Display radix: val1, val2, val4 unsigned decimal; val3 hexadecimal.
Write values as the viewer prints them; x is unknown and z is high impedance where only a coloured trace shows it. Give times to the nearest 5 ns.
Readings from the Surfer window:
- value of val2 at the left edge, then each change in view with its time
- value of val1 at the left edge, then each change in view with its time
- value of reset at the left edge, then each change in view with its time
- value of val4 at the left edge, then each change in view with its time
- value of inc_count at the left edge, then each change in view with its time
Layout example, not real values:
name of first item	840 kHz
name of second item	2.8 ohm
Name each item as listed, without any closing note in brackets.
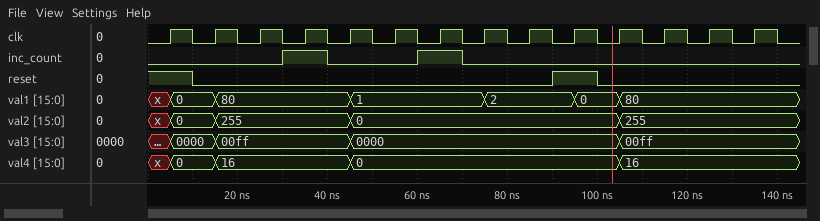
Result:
value of val2 at the left edge, then each change in view with its time	x, 0 at 5 ns, 255 at 15 ns, 0 at 45 ns, 255 at 105 ns
value of val1 at the left edge, then each change in view with its time	x, 0 at 5 ns, 80 at 15 ns, 1 at 45 ns, 2 at 75 ns, 0 at 95 ns, 80 at 105 ns
value of reset at the left edge, then each change in view with its time	1, 0 at 10 ns, 1 at 90 ns, 0 at 100 ns
value of val4 at the left edge, then each change in view with its time	x, 0 at 5 ns, 16 at 15 ns, 0 at 45 ns, 16 at 105 ns
value of inc_count at the left edge, then each change in view with its time	0, 1 at 30 ns, 0 at 40 ns, 1 at 60 ns, 0 at 70 ns
